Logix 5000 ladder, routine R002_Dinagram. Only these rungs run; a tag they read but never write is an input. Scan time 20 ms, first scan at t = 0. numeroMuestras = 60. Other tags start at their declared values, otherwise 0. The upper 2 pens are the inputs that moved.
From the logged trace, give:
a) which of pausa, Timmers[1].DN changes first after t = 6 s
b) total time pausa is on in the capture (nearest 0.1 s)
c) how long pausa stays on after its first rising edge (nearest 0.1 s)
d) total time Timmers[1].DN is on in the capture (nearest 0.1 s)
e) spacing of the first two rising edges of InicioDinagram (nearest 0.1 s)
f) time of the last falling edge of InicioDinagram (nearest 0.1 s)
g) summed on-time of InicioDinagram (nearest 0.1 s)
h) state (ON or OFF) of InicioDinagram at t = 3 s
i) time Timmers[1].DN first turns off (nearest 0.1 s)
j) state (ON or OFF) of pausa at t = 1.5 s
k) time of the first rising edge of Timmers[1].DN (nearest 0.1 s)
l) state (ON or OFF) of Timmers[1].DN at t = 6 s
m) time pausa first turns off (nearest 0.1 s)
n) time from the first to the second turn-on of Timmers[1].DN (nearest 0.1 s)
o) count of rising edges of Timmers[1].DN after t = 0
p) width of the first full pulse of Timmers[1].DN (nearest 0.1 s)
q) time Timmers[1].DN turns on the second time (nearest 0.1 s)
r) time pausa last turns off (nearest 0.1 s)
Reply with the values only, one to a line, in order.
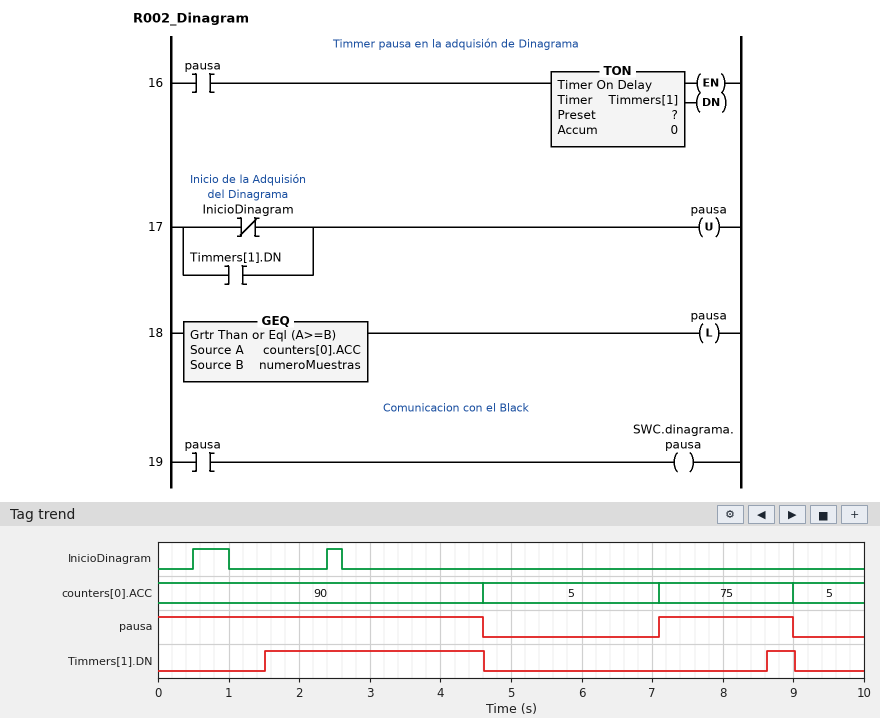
pausa
6.5 s
1.9 s
3.5 s
1.9 s
2.6 s
0.7 s
OFF
4.6 s
ON
1.5 s
OFF
4.6 s
7.1 s
2
3.1 s
8.6 s
9.0 s
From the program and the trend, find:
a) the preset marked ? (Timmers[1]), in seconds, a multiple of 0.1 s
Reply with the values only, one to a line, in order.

1.5 s
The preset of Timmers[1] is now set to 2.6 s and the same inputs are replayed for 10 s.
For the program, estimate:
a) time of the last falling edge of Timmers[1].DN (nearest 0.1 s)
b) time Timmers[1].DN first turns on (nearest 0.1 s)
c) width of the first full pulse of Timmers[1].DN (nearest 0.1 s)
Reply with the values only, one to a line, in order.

4.6 s
2.6 s
2.0 s
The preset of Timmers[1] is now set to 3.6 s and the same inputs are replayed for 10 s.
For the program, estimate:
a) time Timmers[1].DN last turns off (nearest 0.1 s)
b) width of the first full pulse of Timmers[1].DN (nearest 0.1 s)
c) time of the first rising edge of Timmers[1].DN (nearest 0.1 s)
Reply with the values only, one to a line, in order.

4.6 s
1.0 s
3.6 s
